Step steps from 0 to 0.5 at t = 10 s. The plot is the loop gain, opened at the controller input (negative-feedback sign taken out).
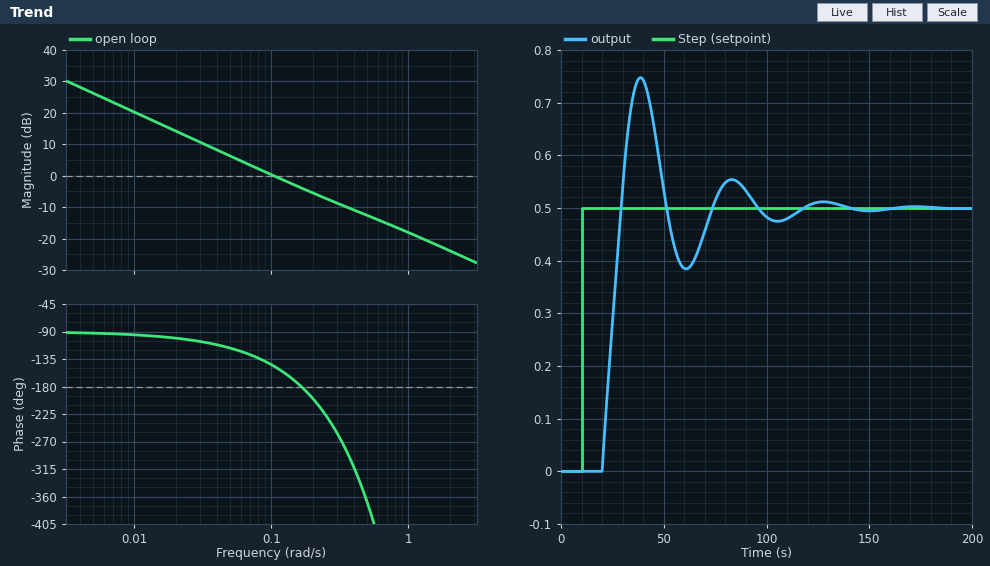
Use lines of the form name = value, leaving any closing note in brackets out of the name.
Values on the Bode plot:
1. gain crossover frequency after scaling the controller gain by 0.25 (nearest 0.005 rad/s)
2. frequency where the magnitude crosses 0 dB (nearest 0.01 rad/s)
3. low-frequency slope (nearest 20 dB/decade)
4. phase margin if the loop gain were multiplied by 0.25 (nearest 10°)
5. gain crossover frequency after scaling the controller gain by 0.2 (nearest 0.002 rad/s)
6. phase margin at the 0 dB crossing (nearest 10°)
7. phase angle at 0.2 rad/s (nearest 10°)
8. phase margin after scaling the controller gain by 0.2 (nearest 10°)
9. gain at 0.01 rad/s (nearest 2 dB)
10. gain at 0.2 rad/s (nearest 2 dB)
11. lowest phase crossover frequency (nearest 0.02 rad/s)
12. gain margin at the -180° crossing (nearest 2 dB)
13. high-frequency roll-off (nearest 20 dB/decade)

gain crossover frequency after scaling the controller gain by 0.25 = 0.025 rad/s
frequency where the magnitude crosses 0 dB = 0.10 rad/s
low-frequency slope = -20 dB/decade
phase margin if the loop gain were multiplied by 0.25 = 80°
gain crossover frequency after scaling the controller gain by 0.2 = 0.020 rad/s
phase margin at the 0 dB crossing = 30°
phase angle at 0.2 rad/s = -200°
phase margin after scaling the controller gain by 0.2 = 80°
gain at 0.01 rad/s = 20 dB
gain at 0.2 rad/s = -6 dB
lowest phase crossover frequency = 0.16 rad/s
gain margin at the -180° crossing = 4 dB
high-frequency roll-off = -20 dB/decade
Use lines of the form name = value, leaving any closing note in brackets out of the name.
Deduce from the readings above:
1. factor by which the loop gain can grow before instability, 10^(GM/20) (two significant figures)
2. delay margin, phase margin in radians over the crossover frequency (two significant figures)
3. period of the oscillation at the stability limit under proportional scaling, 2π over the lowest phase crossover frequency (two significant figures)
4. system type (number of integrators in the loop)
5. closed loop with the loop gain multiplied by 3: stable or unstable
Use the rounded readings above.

factor by which the loop gain can grow before instability, 10^(GM/20) = 1.6
delay margin, phase margin in radians over the crossover frequency = 5.2 s
period of the oscillation at the stability limit under proportional scaling, 2π over the lowest phase crossover frequency = 39 s
system type = 1
closed loop with the loop gain multiplied by 3: stable or unstable = unstable
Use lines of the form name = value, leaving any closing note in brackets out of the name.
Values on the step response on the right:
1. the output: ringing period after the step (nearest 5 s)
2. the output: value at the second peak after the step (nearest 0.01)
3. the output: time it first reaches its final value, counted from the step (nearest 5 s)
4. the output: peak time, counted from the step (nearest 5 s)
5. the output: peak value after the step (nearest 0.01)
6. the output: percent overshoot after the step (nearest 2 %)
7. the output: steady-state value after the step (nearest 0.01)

the output: ringing period after the step = 45 s
the output: value at the second peak after the step = 0.55
the output: time it first reaches its final value, counted from the step = 20 s
the output: peak time, counted from the step = 30 s
the output: peak value after the step = 0.75
the output: percent overshoot after the step = 50 %
the output: steady-state value after the step = 0.50
